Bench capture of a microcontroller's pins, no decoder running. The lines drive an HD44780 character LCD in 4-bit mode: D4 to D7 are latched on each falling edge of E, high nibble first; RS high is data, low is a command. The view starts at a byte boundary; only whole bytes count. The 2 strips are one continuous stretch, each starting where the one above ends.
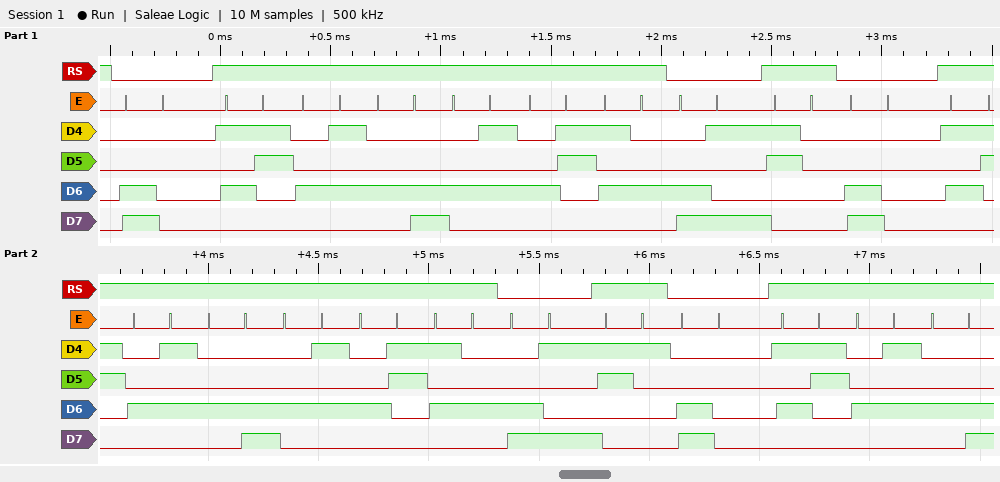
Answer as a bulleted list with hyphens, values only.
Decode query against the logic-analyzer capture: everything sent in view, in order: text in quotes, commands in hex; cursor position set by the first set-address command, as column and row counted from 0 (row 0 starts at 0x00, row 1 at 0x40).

- 0xC0 "SELECT" 0xC9 "0" 0xC0 "SELECT" 0xC9 "1" 0xC0 "SEL"
- column 0, row 1
